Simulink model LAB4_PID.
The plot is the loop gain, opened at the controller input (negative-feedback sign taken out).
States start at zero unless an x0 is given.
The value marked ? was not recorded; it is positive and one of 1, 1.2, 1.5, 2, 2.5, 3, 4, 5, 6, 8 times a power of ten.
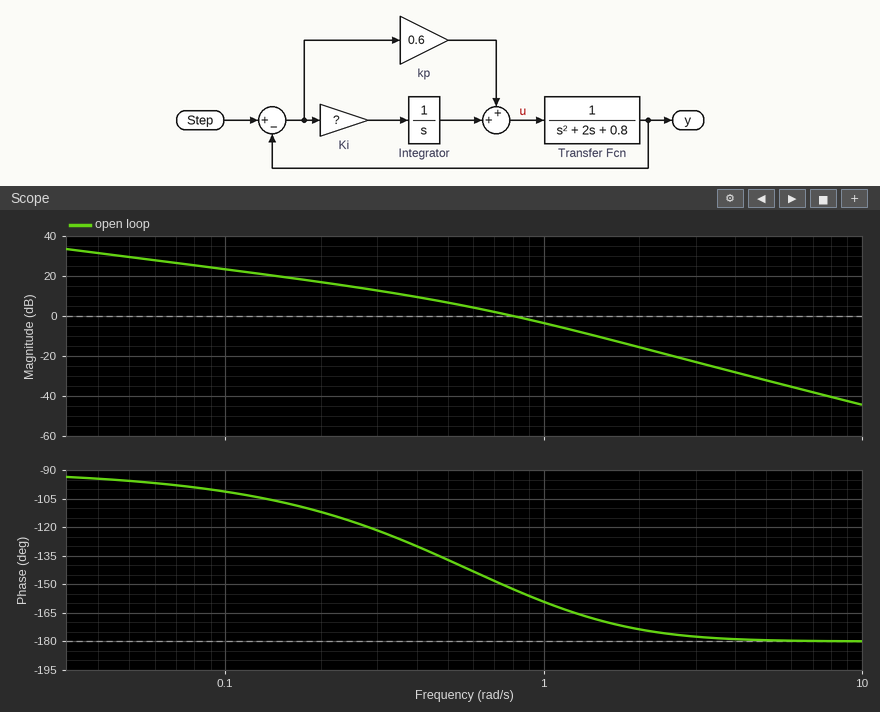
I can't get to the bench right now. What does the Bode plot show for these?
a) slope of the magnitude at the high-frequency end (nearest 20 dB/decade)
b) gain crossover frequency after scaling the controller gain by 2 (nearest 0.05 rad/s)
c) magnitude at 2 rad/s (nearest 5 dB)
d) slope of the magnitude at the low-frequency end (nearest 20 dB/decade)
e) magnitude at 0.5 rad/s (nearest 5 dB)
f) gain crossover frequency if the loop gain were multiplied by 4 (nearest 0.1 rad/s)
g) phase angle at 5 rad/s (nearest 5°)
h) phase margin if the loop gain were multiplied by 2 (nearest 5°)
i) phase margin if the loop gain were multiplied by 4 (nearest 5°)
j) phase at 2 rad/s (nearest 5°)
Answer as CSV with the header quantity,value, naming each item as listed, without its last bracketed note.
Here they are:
quantity,value
slope of the magnitude at the high-frequency end,-40 dB/decade
gain crossover frequency after scaling the controller gain by 2,1.15 rad/s
magnitude at 2 rad/s,-15 dB
slope of the magnitude at the low-frequency end,-20 dB/decade
magnitude at 0.5 rad/s,5 dB
gain crossover frequency if the loop gain were multiplied by 4,1.6 rad/s
phase angle at 5 rad/s,-180°
phase margin if the loop gain were multiplied by 2,15°
phase margin if the loop gain were multiplied by 4,10°
phase at 2 rad/s,-175°
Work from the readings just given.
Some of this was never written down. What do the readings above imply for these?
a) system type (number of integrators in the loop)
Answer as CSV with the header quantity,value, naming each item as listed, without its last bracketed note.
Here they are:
quantity,value
system type,1
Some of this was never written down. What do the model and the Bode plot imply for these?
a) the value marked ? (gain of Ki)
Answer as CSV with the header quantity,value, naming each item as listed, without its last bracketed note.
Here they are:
quantity,value
the value marked ?,1.2
